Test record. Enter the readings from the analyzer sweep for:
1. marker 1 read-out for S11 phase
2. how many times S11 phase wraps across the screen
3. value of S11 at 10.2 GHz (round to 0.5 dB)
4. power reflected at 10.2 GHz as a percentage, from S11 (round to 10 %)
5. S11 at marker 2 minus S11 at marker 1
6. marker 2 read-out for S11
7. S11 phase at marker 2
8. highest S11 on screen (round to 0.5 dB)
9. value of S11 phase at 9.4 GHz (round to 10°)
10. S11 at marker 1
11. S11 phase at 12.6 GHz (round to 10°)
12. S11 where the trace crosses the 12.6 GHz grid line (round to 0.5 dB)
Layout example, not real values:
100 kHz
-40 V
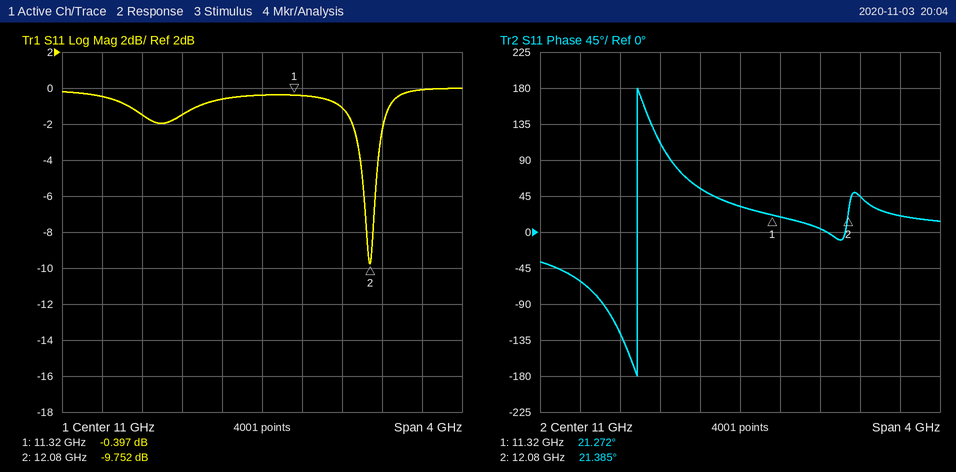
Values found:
21.272°
1
-1.5 dB
70 %
-9.355 dB
-9.752 dB
21.385°
0.0 dB
-60°
-0.397 dB
20°
0.0 dB
